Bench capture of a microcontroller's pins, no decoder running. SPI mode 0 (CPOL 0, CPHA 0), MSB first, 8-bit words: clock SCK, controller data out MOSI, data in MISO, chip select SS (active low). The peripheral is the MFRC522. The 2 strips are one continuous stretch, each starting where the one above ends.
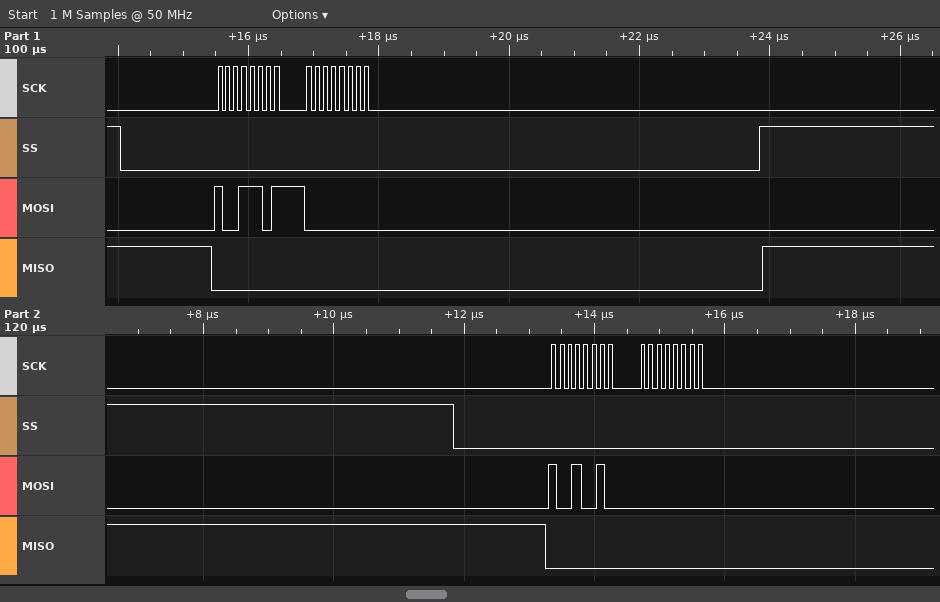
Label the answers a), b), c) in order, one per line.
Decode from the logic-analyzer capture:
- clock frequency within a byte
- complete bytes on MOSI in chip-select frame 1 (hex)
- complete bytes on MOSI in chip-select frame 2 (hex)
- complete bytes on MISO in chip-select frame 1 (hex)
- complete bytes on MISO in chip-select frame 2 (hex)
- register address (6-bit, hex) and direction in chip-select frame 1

a) 8 MHz
b) 9D 00
c) 92 00
d) 00 00
e) 00 00
f) 0x0E read
